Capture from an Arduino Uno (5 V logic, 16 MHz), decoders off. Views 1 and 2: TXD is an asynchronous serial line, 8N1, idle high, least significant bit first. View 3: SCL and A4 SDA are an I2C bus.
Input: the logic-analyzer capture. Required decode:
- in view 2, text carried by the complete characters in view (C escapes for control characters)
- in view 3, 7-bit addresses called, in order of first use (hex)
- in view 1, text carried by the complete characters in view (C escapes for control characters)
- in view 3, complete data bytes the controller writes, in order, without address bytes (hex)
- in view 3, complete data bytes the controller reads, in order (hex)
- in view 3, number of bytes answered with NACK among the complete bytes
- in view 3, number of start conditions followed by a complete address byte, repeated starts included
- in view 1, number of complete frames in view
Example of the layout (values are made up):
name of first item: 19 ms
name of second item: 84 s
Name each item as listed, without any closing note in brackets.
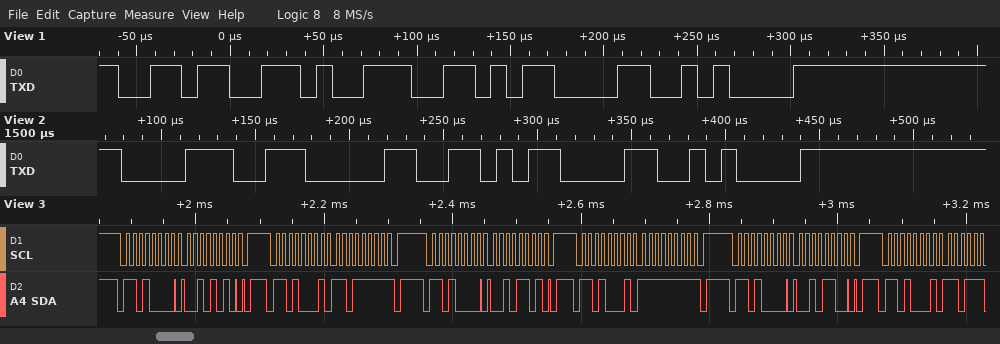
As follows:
in view 2, text carried by the complete characters in view: "80\r\n"
in view 3, 7-bit addresses called, in order of first use: 0x68
in view 1, text carried by the complete characters in view: "69\r\n"
in view 3, complete data bytes the controller writes, in order, without address bytes: 2A 2D 2C
in view 3, complete data bytes the controller reads, in order: DF FF
in view 3, number of bytes answered with NACK among the complete bytes: 2
in view 3, number of start conditions followed by a complete address byte, repeated starts included: 6
in view 1, number of complete frames in view: 4
